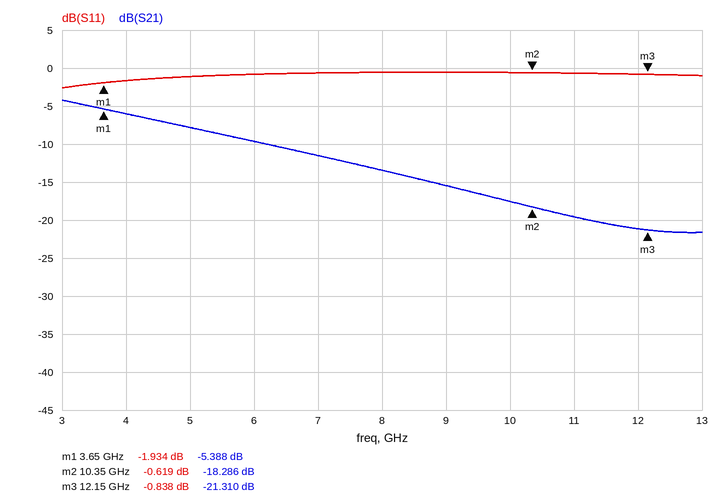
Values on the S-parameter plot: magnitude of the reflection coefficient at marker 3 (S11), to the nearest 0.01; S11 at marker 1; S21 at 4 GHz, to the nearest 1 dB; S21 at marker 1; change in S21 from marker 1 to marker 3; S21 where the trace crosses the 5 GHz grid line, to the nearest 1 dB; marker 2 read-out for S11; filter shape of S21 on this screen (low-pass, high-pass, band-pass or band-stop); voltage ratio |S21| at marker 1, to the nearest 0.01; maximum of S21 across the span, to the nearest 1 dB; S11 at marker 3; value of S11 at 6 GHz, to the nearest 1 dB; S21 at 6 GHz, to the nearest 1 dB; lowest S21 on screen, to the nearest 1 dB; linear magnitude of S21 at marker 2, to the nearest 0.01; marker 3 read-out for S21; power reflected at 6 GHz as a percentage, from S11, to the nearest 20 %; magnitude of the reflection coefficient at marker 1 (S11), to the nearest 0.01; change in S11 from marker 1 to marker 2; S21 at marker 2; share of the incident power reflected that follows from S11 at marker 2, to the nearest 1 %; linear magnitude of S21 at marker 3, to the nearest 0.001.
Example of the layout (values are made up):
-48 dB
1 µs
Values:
0.91
-1.934 dB
-6 dB
-5.388 dB
-15.922 dB
-8 dB
-0.619 dB
low-pass
0.54
-4 dB
-0.838 dB
-1 dB
-10 dB
-22 dB
0.12
-21.310 dB
80 %
0.80
1.315 dB
-18.286 dB
87 %
0.086
